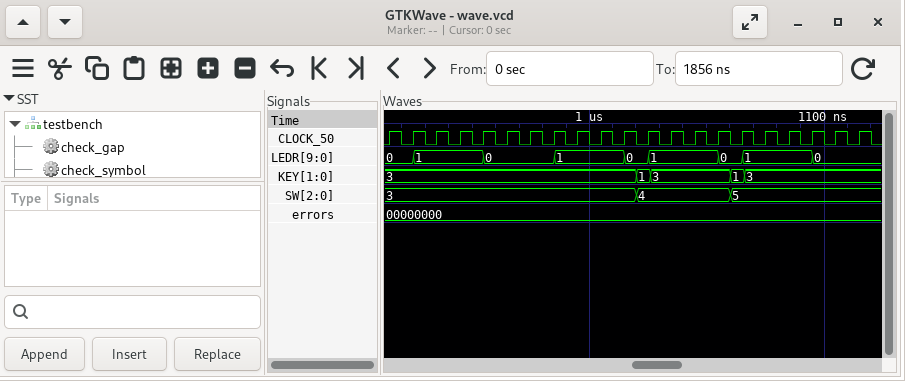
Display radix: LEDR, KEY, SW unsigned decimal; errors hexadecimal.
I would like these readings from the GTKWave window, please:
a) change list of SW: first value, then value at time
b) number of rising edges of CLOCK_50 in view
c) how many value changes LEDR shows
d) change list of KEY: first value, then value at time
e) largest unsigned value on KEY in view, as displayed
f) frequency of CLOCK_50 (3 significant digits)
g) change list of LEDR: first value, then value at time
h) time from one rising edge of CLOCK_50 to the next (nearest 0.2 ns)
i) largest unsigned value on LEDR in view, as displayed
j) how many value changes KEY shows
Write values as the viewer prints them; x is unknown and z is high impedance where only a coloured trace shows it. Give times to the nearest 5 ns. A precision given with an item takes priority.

3, 4 at 1020 ns, 5 at 1060 ns
21
8
3, 1 at 1020 ns, 3 at 1025 ns, 1 at 1060 ns, 3 at 1065 ns
3
100 MHz
0, 1 at 925 ns, 0 at 955 ns, 1 at 985 ns, 0 at 1015 ns, 1 at 1025 ns, 0 at 1055 ns, 1 at 1065 ns, 0 at 1095 ns
10 ns
1
4
